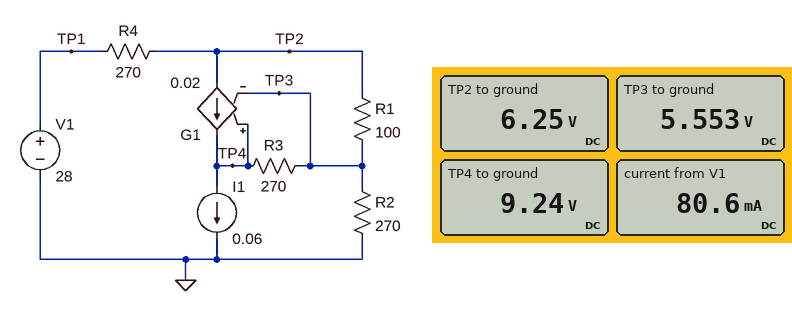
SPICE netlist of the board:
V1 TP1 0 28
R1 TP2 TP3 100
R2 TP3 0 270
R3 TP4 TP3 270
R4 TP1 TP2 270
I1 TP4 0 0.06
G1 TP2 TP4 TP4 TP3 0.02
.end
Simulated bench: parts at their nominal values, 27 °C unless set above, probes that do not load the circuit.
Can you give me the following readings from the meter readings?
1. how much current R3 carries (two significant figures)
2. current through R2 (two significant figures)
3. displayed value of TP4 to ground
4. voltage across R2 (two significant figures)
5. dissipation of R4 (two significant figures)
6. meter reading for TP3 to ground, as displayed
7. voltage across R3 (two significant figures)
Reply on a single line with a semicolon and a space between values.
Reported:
14 mA; 21 mA; 9.24 V; 5.6 V; 1.8 W; 5.553 V; 3.7 V
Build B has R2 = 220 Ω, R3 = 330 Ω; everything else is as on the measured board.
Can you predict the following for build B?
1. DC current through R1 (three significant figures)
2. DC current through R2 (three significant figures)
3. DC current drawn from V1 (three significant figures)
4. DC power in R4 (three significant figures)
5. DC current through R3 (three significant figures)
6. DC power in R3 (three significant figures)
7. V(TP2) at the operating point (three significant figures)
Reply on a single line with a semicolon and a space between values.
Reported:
11.1 mA; 21.8 mA; 81.8 mA; 1.81 W; 10.7 mA; 37.9 mW; 5.91 V
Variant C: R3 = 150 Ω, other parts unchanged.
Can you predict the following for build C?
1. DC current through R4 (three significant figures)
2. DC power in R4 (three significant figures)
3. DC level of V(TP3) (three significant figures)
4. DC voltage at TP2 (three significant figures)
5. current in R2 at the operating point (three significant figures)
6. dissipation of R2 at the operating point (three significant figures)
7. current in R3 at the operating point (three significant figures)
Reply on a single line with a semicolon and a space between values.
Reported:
83.1 mA; 1.87 W; 6.24 V; 5.56 V; 23.1 mA; 144 mW; 30.0 mA
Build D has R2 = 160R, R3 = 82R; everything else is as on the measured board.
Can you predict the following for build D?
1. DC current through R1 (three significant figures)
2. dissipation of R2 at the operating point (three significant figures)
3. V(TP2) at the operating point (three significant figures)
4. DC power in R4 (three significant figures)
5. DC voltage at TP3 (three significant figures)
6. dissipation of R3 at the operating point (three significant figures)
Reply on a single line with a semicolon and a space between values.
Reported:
53.8 mA; 255 mW; 1.01 V; 2.70 W; 6.39 V; 721 mW
